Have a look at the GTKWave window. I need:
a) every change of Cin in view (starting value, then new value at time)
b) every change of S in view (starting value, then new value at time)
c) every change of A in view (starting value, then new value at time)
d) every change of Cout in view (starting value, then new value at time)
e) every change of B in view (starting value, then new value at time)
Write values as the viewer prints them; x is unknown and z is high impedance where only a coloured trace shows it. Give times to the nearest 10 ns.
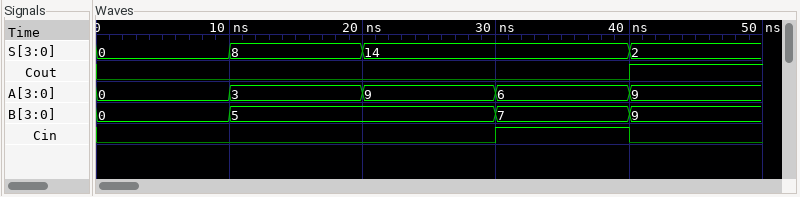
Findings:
0, 1 at 30 ns, 0 at 40 ns
0, 8 at 10 ns, 14 at 20 ns, 2 at 40 ns
0, 3 at 10 ns, 9 at 20 ns, 6 at 30 ns, 9 at 40 ns
0, 1 at 40 ns
0, 5 at 10 ns, 7 at 30 ns, 9 at 40 ns
